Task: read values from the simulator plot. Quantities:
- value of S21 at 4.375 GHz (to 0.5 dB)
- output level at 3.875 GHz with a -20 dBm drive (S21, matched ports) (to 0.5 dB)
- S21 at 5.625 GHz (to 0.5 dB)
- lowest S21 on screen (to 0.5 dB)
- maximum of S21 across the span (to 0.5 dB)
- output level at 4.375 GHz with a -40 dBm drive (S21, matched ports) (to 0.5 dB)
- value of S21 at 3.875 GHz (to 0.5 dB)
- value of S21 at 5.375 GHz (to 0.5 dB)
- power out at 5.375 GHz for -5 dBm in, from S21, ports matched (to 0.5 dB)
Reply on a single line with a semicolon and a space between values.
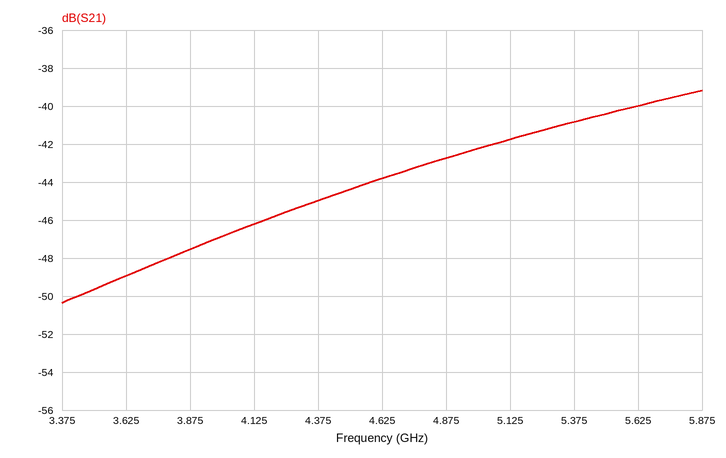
-45.0 dB; -67.5 dBm; -40.0 dB; -50.5 dB; -39.0 dB; -85.0 dBm; -47.5 dB; -41.0 dB; -46.0 dBm
